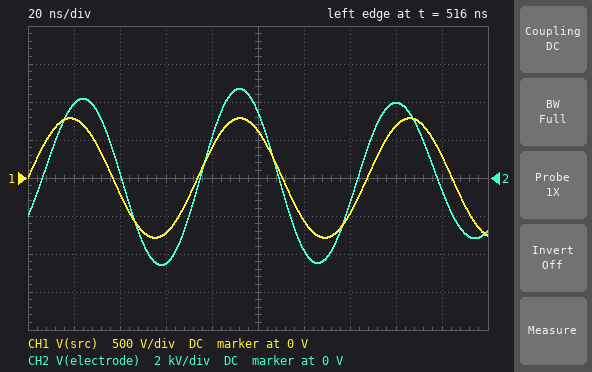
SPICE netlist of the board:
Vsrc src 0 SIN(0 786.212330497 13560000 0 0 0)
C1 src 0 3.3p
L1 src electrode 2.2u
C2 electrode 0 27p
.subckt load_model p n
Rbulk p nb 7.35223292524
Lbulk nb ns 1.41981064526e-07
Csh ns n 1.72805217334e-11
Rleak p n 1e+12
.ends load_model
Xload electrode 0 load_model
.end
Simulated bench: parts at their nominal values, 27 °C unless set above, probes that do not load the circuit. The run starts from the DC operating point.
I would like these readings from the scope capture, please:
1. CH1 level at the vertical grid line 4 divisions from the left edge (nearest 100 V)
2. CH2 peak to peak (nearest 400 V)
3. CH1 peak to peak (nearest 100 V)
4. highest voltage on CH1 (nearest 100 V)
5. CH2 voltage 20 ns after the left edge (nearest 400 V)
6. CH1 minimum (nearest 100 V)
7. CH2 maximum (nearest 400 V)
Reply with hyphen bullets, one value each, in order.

- 400 V
- 9.2 kV
- 1.6 kV
- 800 V
- 4.0 kV
- -800 V
- 4.8 kV
